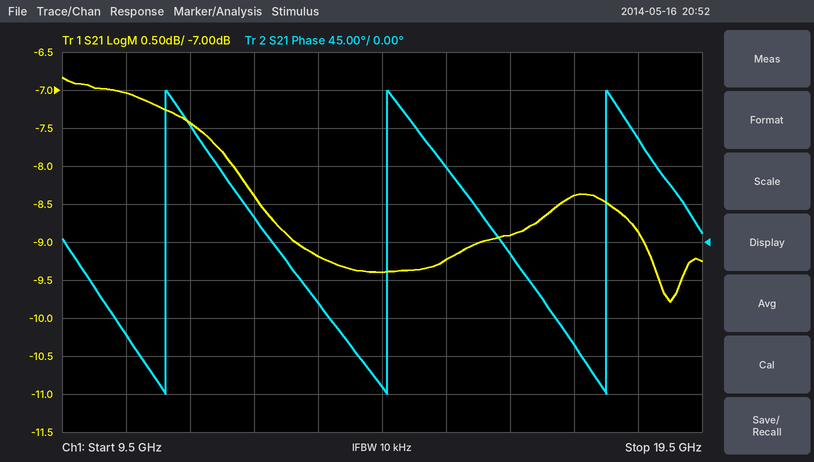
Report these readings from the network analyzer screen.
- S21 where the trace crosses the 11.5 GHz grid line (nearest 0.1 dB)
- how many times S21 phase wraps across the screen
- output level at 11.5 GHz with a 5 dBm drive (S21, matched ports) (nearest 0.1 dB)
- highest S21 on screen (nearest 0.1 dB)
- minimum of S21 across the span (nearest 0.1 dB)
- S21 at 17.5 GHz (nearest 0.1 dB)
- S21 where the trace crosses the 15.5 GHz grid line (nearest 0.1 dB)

-7.4 dB
3
-2.4 dBm
-6.8 dB
-9.8 dB
-8.4 dB
-9.2 dB
